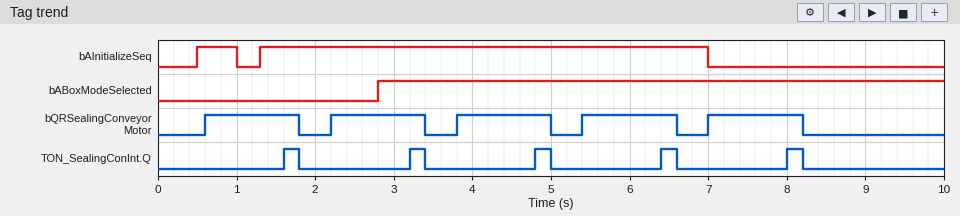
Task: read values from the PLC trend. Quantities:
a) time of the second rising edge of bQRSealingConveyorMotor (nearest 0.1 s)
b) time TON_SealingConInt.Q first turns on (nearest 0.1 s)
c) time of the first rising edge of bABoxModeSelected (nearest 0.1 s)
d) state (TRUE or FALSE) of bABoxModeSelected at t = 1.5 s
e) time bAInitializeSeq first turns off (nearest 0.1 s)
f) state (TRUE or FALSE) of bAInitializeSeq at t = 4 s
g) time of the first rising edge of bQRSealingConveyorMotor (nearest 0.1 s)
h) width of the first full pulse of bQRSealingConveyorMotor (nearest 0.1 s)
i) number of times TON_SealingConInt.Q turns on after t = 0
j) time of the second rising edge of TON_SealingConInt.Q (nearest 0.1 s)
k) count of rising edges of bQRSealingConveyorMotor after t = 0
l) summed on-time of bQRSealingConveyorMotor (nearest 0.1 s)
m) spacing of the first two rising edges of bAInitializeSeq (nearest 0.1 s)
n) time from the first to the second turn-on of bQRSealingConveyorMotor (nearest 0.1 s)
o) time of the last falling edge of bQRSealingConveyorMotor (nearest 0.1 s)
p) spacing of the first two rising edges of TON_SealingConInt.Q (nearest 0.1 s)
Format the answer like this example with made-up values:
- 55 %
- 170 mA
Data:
- 2.2 s
- 1.6 s
- 2.8 s
- FALSE
- 1.0 s
- TRUE
- 0.6 s
- 1.2 s
- 5
- 3.2 s
- 5
- 6.0 s
- 0.8 s
- 1.6 s
- 8.2 s
- 1.6 s
